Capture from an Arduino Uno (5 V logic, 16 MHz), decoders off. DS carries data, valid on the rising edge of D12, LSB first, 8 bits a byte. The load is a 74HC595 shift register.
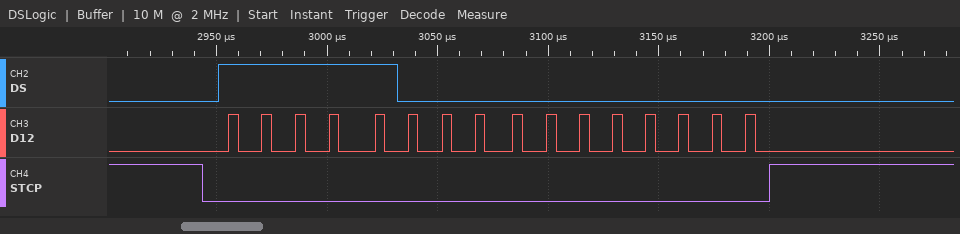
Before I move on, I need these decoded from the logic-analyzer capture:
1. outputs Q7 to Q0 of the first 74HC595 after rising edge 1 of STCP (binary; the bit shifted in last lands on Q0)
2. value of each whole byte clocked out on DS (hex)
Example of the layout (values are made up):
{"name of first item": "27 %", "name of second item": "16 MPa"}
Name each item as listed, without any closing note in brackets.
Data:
{"outputs Q7 to Q0 of the first 74HC595 after rising edge 1 of STCP": "00000000", "value of each whole byte clocked out on DS": "1F 00"}
